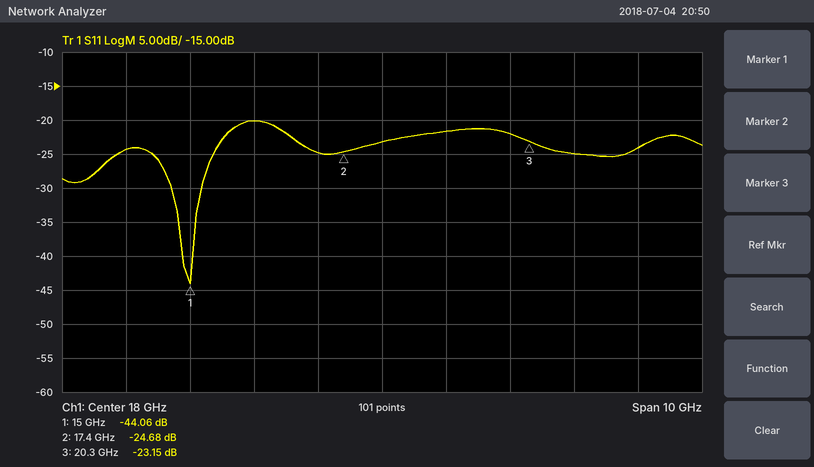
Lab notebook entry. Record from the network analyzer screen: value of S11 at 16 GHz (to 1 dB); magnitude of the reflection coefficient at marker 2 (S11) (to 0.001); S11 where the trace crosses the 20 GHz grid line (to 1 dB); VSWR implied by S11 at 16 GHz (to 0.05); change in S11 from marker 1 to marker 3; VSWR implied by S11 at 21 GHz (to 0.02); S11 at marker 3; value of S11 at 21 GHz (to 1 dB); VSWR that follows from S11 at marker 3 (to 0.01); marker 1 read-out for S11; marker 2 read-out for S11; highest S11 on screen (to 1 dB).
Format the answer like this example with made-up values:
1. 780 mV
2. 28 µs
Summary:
1. -20 dB
2. 0.058
3. -22 dB
4. 1.20
5. 20.91 dB
6. 1.12
7. -23.15 dB
8. -25 dB
9. 1.15
10. -44.06 dB
11. -24.68 dB
12. -20 dB
